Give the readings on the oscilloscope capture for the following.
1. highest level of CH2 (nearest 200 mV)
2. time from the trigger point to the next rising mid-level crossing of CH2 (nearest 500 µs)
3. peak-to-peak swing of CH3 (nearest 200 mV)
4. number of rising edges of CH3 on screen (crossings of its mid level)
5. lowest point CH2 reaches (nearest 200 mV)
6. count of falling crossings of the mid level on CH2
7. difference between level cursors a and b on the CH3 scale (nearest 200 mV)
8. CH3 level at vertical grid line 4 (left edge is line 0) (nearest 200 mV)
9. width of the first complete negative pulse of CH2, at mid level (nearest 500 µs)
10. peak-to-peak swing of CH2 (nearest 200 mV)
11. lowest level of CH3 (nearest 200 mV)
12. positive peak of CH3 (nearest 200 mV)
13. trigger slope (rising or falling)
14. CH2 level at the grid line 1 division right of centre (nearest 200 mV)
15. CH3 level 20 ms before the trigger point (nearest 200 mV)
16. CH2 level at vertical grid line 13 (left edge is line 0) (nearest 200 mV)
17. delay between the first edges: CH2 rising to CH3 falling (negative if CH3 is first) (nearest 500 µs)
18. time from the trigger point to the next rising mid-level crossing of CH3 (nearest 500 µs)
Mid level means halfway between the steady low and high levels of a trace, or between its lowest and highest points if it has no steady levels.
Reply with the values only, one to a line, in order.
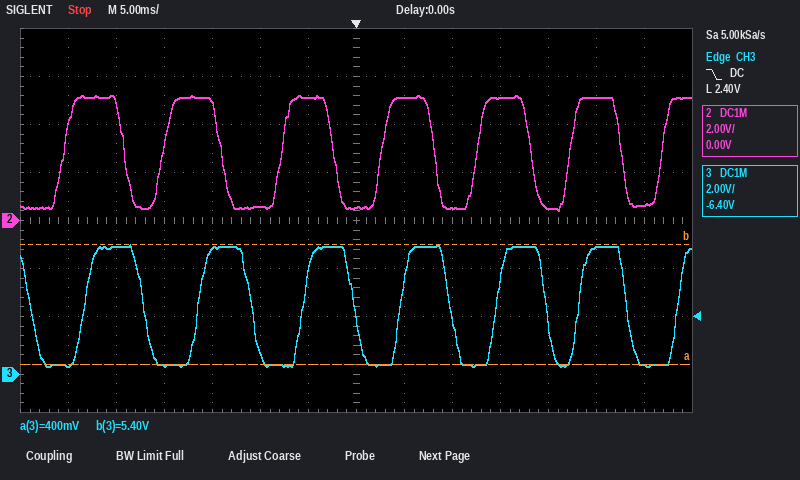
5.2 V
2.5 ms
5.0 V
7
400 mV
6
5.0 V
5.2 V
4.0 ms
4.8 V
400 mV
5.4 V
falling
5.2 V
400 mV
600 mV
-3.5 ms
4.5 ms
